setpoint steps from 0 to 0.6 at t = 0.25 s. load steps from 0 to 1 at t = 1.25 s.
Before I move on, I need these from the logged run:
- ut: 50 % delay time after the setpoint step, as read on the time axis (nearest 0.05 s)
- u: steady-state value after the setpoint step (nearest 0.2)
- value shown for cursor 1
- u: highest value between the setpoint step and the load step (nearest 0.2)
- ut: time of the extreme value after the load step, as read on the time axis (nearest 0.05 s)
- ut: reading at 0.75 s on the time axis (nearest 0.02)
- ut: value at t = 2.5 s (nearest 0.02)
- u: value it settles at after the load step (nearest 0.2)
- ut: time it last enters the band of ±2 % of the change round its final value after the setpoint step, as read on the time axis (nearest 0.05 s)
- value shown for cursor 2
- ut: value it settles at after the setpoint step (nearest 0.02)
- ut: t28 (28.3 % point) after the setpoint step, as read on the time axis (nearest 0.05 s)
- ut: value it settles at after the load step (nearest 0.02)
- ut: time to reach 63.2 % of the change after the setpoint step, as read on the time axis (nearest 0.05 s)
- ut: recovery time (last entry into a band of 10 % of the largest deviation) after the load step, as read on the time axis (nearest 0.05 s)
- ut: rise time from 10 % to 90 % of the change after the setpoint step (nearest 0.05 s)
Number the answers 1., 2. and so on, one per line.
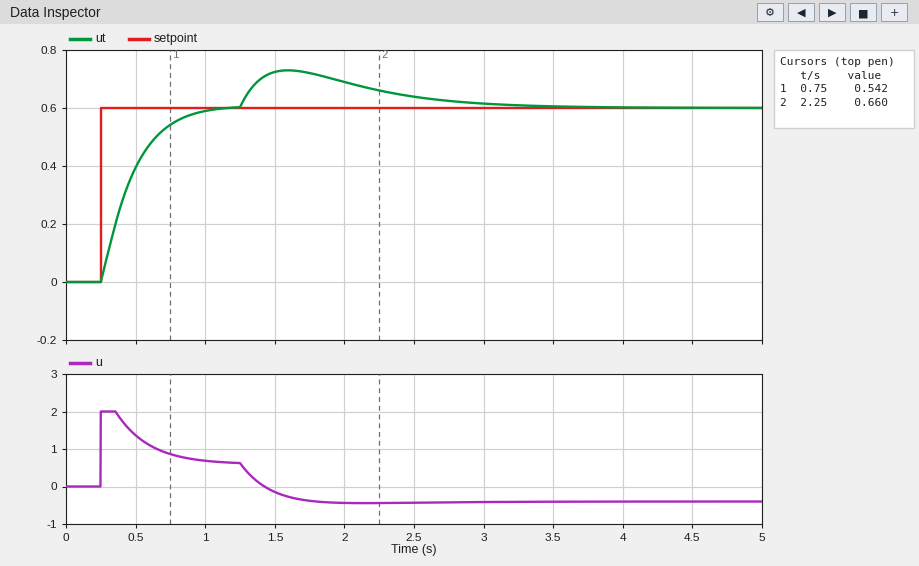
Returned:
1. 0.40 s
2. 0.6
3. 0.542
4. 2.0
5. 1.60 s
6. 0.54
7. 0.64
8. -0.4
9. 1.00 s
10. 0.660
11. 0.60
12. 0.35 s
13. 0.60
14. 0.50 s
15. 3.10 s
16. 0.45 s
